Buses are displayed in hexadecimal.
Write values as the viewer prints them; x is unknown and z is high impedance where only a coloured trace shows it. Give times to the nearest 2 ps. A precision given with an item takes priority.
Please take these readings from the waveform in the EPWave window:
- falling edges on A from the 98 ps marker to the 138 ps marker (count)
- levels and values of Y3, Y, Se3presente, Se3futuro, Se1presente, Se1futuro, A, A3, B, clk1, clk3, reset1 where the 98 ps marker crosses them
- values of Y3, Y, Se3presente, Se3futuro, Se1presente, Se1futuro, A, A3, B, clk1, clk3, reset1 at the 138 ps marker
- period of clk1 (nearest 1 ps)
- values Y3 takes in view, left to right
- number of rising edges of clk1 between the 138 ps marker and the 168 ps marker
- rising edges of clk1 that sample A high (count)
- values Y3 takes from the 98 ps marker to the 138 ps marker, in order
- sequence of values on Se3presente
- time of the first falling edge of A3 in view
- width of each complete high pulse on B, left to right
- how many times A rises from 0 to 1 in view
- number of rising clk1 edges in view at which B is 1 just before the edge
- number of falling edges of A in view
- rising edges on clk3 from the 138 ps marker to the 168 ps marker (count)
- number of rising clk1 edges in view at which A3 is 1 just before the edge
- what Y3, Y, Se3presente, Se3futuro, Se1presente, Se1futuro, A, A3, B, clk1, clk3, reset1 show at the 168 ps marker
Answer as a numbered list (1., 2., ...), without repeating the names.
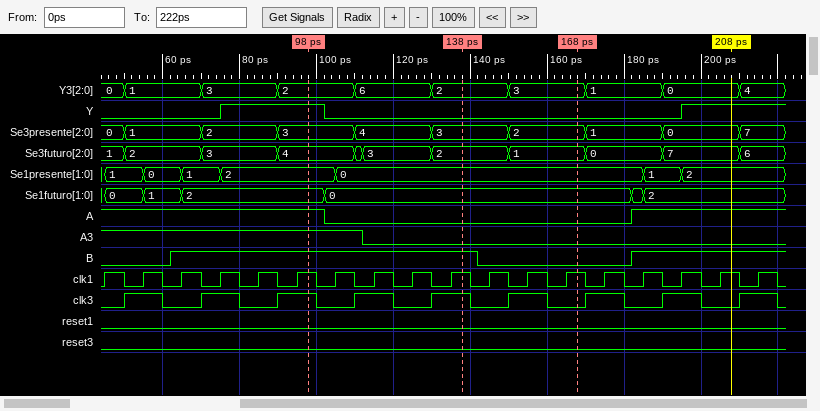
1. 1
2. Y3=2, Y=1, Se3presente=3, Se3futuro=4, Se1presente=2, Se1futuro=2, A=1, A3=1, B=1, clk1=1, clk3=1, reset1=0
3. Y3=2, Y=0, Se3presente=3, Se3futuro=2, Se1presente=0, Se1futuro=0, A=0, A3=0, B=1, clk1=1, clk3=1, reset1=0
4. 10 ps
5. 0, 1, 3, 2, 6, 2, 3, 1, 0, 4
6. 3
7. 10
8. 2, 6, 2
9. 0, 1, 2, 3, 4, 3, 2, 1, 0, 7
10. 112 ps
11. 80 ps
12. 1
13. 12
14. 1
15. 1
16. 7
17. Y3=3, Y=0, Se3presente=2, Se3futuro=1, Se1presente=0, Se1futuro=0, A=0, A3=0, B=0, clk1=1, clk3=0, reset1=0
